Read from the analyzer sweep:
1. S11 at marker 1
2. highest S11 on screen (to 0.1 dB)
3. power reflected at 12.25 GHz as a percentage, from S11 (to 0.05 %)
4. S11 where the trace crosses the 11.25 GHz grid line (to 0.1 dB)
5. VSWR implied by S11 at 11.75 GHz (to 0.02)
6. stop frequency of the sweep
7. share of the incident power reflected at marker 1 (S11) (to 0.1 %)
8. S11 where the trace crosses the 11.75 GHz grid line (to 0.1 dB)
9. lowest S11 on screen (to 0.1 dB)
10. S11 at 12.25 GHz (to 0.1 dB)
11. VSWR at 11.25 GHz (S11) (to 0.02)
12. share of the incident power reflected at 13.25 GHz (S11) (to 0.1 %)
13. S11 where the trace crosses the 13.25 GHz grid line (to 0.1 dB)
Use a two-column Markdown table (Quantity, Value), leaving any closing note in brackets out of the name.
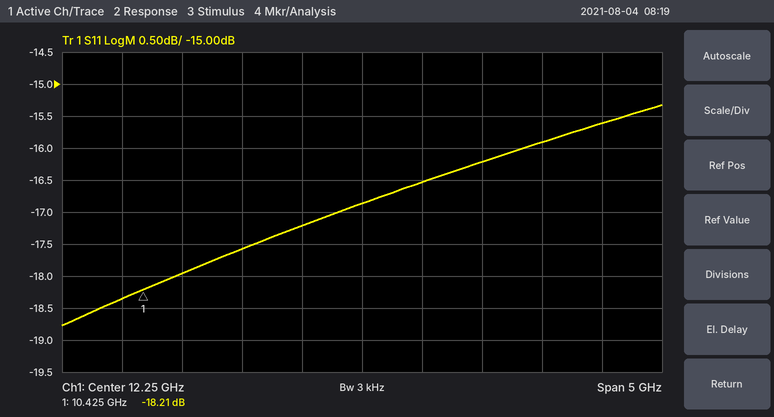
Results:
| Quantity | Value |
|---|---|
| S11 at marker 1 | -18.21 dB |
| highest S11 on screen | -15.3 dB |
| power reflected at 12.25 GHz as a percentage, from S11 | 2.05 % |
| S11 where the trace crosses the 11.25 GHz grid line | -17.6 dB |
| VSWR implied by S11 at 11.75 GHz | 1.32 |
| stop frequency of the sweep | 14.75 GHz |
| share of the incident power reflected at marker 1 (S11) | 1.5 % |
| S11 where the trace crosses the 11.75 GHz grid line | -17.2 dB |
| lowest S11 on screen | -18.8 dB |
| S11 at 12.25 GHz | -16.9 dB |
| VSWR at 11.25 GHz (S11) | 1.30 |
| share of the incident power reflected at 13.25 GHz (S11) | 2.4 % |
| S11 where the trace crosses the 13.25 GHz grid line | -16.2 dB |
